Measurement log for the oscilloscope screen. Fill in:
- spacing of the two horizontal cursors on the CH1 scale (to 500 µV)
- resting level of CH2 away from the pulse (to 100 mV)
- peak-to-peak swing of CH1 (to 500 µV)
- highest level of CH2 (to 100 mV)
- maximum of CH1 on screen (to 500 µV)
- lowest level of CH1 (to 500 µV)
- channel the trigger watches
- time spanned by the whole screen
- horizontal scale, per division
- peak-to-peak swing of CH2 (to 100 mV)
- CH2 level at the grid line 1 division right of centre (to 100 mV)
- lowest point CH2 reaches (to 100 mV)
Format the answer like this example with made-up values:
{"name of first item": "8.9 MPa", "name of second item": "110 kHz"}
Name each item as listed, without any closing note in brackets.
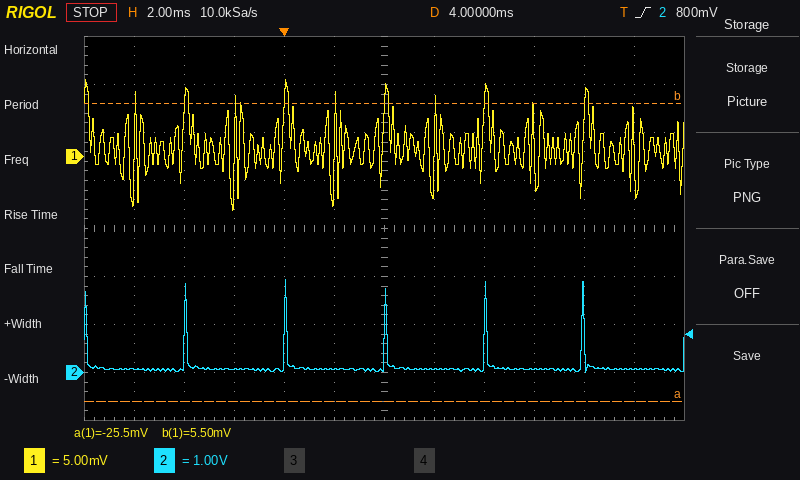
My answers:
{"spacing of the two horizontal cursors on the CH1 scale": "31.0 mV", "resting level of CH2 away from the pulse": "100 mV", "peak-to-peak swing of CH1": "13.5 mV", "highest level of CH2": "1.9 V", "maximum of CH1 on screen": "8.0 mV", "lowest level of CH1": "-5.5 mV", "channel the trigger watches": "CH2", "time spanned by the whole screen": "24 ms", "horizontal scale, per division": "2 ms", "peak-to-peak swing of CH2": "1.9 V", "CH2 level at the grid line 1 division right of centre": "100 mV", "lowest point CH2 reaches": "0.0 V"}
